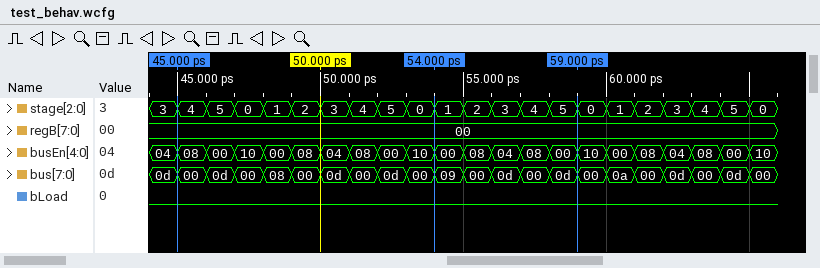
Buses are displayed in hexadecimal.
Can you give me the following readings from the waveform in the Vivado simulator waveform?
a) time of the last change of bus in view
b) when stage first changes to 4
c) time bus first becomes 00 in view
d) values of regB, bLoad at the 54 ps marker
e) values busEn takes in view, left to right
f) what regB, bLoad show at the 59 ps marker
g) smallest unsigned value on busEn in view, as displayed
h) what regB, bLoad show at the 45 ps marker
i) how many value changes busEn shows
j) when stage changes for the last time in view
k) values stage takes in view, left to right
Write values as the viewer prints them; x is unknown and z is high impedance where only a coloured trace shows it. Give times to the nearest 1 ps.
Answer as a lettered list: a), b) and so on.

a) 65 ps
b) 45 ps
c) 45 ps
d) regB=00, bLoad=0
e) 04, 08, 00, 10, 00, 08, 04, 08, 00, 10, 00, 08, 04, 08, 00, 10, 00, 08, 04, 08, 00, 10
f) regB=00, bLoad=0
g) 00
h) regB=00, bLoad=0
i) 21
j) 65 ps
k) 3, 4, 5, 0, 1, 2, 3, 4, 5, 0, 1, 2, 3, 4, 5, 0, 1, 2, 3, 4, 5, 0
